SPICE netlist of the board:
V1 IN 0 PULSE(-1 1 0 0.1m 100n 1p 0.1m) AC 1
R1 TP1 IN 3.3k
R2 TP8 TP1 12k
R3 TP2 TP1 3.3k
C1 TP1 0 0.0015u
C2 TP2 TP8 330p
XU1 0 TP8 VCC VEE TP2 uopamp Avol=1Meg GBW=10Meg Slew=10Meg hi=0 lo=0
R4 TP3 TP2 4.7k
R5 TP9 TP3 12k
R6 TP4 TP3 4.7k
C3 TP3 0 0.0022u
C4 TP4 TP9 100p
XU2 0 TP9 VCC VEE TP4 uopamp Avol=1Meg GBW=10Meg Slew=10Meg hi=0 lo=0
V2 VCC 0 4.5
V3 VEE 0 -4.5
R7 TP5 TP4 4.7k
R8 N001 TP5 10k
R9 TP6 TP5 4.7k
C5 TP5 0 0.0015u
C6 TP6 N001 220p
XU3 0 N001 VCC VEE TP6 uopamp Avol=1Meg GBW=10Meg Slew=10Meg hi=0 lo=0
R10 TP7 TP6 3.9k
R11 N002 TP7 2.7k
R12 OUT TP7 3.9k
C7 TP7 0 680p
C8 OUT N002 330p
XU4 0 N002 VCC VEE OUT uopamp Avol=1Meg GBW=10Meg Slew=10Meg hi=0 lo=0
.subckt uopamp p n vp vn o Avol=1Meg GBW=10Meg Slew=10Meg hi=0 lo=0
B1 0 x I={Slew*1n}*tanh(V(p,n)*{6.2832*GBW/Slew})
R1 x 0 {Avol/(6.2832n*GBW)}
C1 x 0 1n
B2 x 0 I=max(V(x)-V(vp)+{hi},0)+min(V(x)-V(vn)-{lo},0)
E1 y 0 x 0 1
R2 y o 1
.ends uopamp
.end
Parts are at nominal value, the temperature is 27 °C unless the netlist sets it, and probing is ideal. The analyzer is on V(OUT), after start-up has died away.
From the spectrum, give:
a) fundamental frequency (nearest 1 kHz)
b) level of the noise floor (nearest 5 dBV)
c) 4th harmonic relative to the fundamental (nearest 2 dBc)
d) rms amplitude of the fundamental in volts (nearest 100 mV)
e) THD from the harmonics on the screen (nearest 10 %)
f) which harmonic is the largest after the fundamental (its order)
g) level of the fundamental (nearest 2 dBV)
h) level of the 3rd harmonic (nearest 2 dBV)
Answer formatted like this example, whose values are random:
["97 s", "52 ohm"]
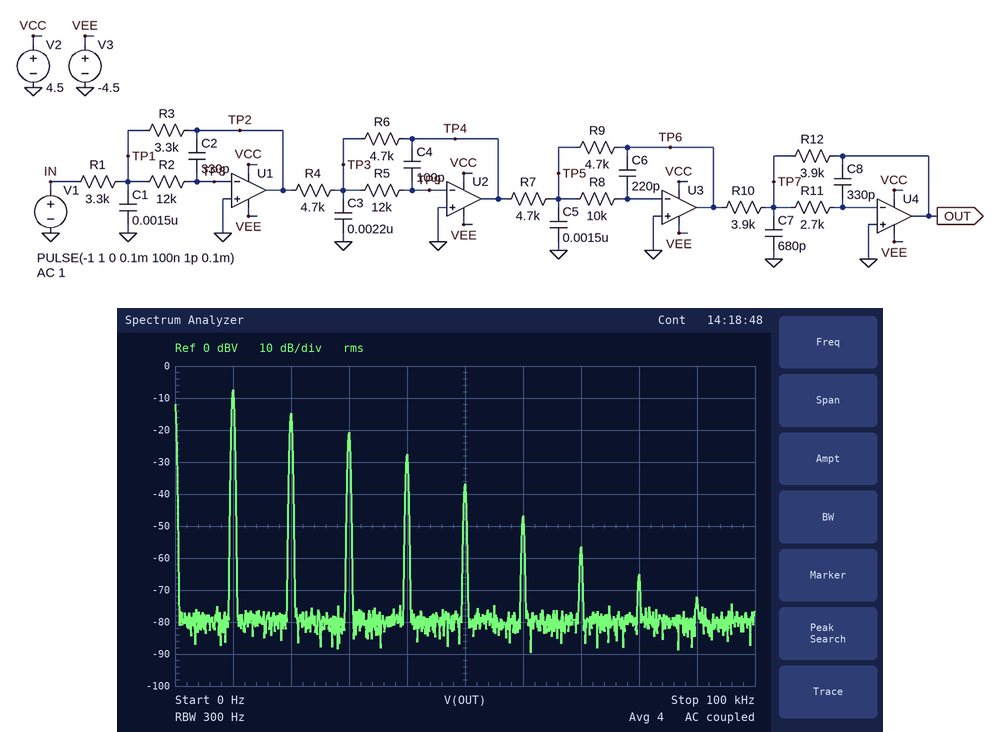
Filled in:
["10 kHz", "-80 dBV", "-20 dBc", "400 mV", "50 %", "2", "-8 dBV", "-20 dBV"]
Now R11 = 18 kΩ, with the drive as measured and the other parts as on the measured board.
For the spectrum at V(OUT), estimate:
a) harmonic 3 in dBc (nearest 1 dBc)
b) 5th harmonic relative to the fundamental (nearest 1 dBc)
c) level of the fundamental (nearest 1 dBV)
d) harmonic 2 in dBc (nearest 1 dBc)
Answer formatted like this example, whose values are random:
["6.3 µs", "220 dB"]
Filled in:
["-19 dBc", "-38 dBc", "-9 dBV", "-10 dBc"]
